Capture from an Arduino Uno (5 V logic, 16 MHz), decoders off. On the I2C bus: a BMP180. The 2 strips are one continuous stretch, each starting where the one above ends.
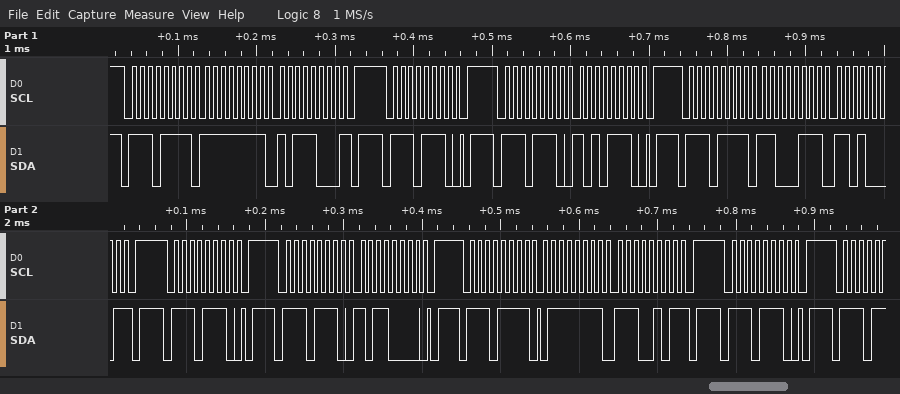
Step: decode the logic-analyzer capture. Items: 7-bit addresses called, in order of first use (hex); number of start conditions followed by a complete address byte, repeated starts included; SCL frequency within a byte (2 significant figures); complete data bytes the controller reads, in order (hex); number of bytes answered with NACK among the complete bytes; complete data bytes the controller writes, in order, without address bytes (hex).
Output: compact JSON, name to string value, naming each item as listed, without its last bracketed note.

{"7-bit addresses called, in order of first use": "0x77", "number of start conditions followed by a complete address byte, repeated starts included": "8", "SCL frequency within a byte": "100 kHz", "complete data bytes the controller reads, in order": "FF B8 C7 D1 7F E5", "number of bytes answered with NACK among the complete bytes": "3", "complete data bytes the controller writes, in order, without address bytes": "AE B0"}
